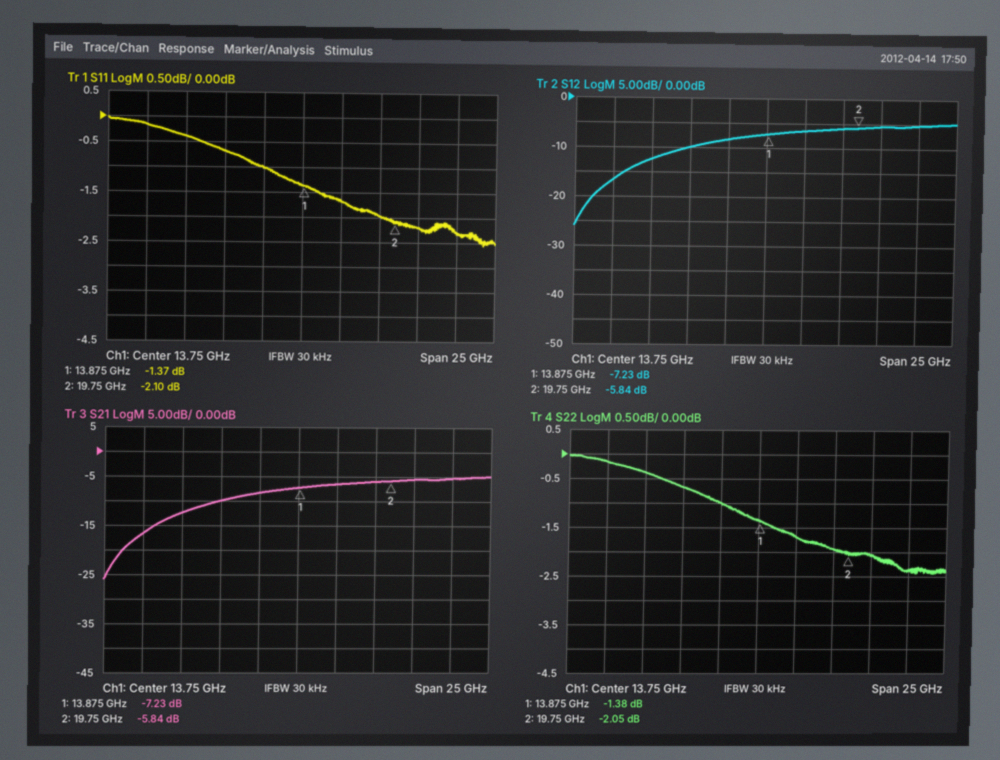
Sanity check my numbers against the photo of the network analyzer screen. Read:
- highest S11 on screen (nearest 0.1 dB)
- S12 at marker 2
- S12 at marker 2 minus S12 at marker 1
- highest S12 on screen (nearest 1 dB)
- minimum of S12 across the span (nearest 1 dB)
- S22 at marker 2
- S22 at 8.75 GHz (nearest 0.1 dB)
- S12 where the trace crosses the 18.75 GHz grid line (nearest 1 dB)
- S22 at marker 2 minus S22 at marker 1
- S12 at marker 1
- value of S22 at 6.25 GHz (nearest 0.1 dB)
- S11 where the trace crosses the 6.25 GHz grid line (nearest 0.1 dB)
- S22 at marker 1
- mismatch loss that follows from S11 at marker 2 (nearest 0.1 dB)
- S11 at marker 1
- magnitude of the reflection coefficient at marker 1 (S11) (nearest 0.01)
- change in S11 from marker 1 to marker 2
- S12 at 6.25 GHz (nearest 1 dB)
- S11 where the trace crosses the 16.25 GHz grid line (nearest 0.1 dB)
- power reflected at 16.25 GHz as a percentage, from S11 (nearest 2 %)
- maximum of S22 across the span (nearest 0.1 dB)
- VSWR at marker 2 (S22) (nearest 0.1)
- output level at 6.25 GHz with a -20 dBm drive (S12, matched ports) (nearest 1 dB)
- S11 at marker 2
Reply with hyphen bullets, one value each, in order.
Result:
- 0.0 dB
- -5.84 dB
- 1.39 dB
- -5 dB
- -26 dB
- -2.05 dB
- -0.7 dB
- -6 dB
- -0.67 dB
- -7.23 dB
- -0.4 dB
- -0.4 dB
- -1.38 dB
- 4.2 dB
- -1.37 dB
- 0.85
- -0.73 dB
- -12 dB
- -1.7 dB
- 68 %
- 0.0 dB
- 8.5
- -32 dBm
- -2.10 dB
